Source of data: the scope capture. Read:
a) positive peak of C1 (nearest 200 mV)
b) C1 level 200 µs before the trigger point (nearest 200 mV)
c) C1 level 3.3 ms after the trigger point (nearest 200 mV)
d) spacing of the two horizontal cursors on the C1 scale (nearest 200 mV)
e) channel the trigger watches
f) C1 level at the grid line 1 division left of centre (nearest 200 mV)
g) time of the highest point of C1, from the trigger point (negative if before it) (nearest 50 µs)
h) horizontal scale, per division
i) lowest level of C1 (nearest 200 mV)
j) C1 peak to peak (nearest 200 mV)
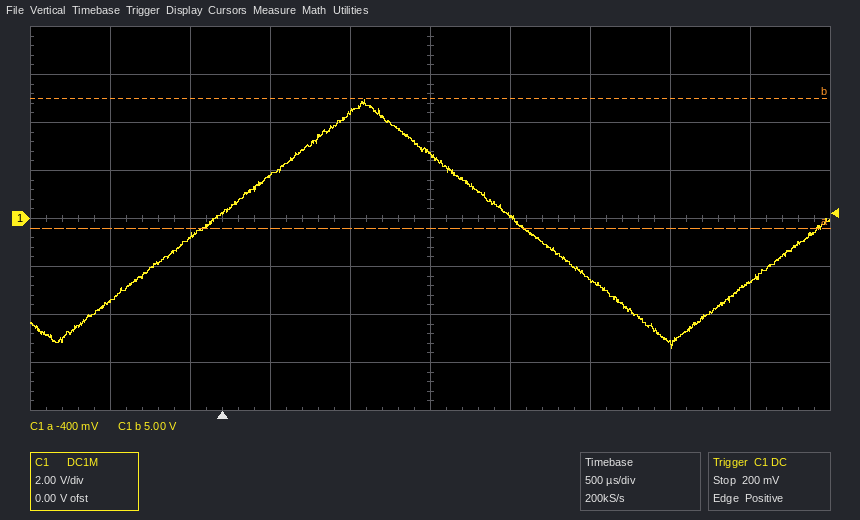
5.0 V
-800 mV
-2.6 V
5.4 V
C1
4.4 V
+900 µs
500 µs
-5.4 V
10.4 V
